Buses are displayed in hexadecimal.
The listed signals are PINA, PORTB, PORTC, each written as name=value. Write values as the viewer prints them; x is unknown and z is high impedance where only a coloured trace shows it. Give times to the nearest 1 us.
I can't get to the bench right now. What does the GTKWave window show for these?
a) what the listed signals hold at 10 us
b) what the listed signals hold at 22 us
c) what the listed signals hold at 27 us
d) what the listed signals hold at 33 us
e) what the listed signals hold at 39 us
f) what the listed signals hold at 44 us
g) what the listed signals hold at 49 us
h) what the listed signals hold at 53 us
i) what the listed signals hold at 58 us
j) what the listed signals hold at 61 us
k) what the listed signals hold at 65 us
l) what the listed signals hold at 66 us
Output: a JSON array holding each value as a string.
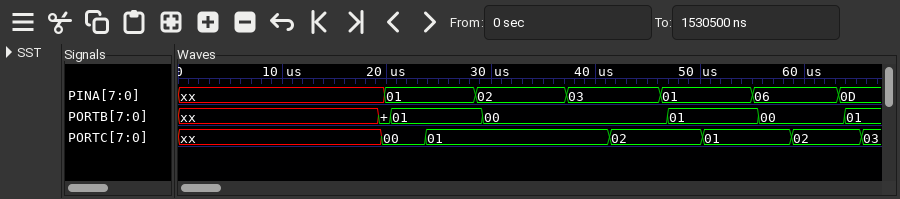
["PINA=xx, PORTB=xx, PORTC=xx", "PINA=01, PORTB=01, PORTC=00", "PINA=01, PORTB=01, PORTC=01", "PINA=02, PORTB=00, PORTC=01", "PINA=03, PORTB=00, PORTC=01", "PINA=03, PORTB=00, PORTC=02", "PINA=01, PORTB=01, PORTC=02", "PINA=01, PORTB=01, PORTC=01", "PINA=06, PORTB=00, PORTC=01", "PINA=06, PORTB=00, PORTC=02", "PINA=0D, PORTB=01, PORTC=02", "PINA=0D, PORTB=01, PORTC=03"]
